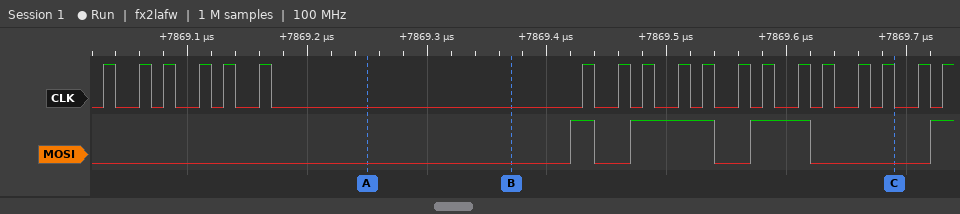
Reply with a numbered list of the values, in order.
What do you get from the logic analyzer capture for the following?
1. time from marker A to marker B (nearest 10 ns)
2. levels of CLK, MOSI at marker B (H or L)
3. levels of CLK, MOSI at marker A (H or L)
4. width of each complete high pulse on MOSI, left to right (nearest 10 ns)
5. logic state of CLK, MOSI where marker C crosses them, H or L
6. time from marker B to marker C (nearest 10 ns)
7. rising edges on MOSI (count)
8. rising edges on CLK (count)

1. 120 ns
2. CLK=L, MOSI=L
3. CLK=L, MOSI=L
4. 20 ns, 70 ns, 50 ns
5. CLK=L, MOSI=L
6. 320 ns
7. 4
8. 19
